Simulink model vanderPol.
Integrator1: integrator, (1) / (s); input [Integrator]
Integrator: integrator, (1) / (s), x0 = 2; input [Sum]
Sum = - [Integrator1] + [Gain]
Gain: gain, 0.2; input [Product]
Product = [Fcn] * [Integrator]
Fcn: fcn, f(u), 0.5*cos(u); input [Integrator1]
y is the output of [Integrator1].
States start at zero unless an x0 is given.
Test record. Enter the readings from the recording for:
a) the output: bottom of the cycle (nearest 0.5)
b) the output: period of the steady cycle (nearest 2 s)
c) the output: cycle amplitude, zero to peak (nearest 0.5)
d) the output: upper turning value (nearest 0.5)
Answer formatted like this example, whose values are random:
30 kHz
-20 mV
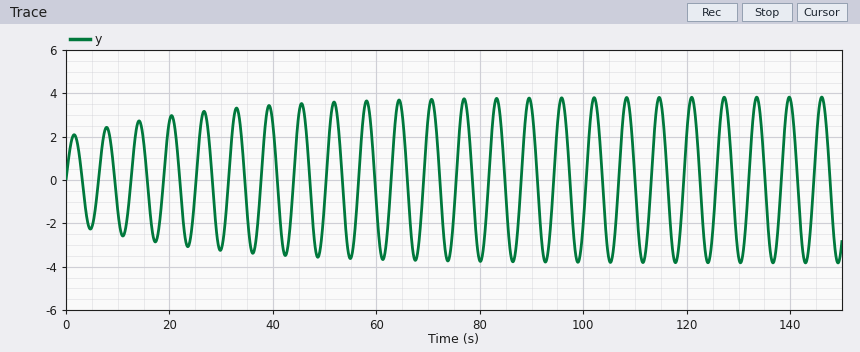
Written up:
-4.0
6 s
4.0
4.0
